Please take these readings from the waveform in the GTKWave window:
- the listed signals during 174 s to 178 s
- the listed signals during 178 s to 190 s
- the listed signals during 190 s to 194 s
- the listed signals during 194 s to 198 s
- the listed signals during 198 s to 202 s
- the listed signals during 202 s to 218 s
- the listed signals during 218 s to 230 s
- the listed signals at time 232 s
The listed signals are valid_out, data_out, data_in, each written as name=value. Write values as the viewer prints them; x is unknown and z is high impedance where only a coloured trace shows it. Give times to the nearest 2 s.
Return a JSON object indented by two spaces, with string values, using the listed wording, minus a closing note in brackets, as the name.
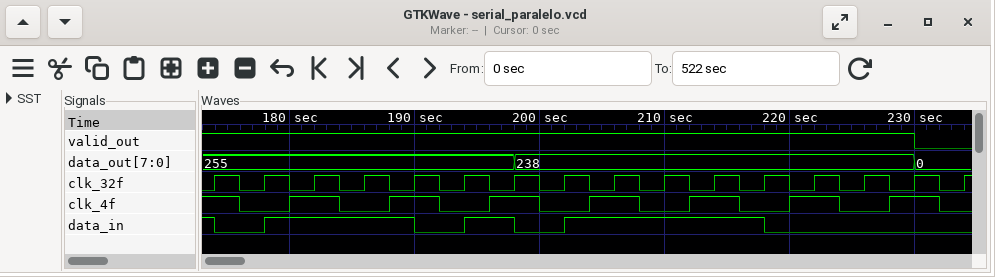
{
  "the listed signals during 174 s to 178 s": "valid_out=1, data_out=255, data_in=0",
  "the listed signals during 178 s to 190 s": "valid_out=1, data_out=255, data_in=1",
  "the listed signals during 190 s to 194 s": "valid_out=1, data_out=255, data_in=0",
  "the listed signals during 194 s to 198 s": "valid_out=1, data_out=255, data_in=1",
  "the listed signals during 198 s to 202 s": "valid_out=1, data_out=238, data_in=0",
  "the listed signals during 202 s to 218 s": "valid_out=1, data_out=238, data_in=1",
  "the listed signals during 218 s to 230 s": "valid_out=1, data_out=238, data_in=0",
  "the listed signals at time 232 s": "valid_out=0, data_out=0, data_in=0"
}
